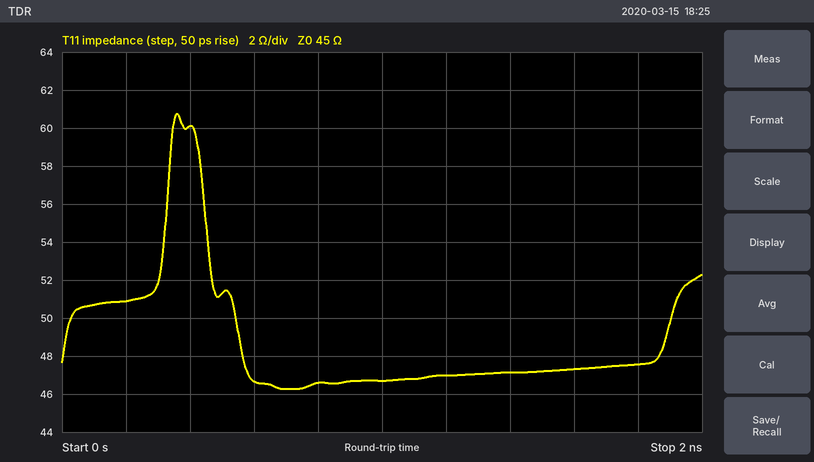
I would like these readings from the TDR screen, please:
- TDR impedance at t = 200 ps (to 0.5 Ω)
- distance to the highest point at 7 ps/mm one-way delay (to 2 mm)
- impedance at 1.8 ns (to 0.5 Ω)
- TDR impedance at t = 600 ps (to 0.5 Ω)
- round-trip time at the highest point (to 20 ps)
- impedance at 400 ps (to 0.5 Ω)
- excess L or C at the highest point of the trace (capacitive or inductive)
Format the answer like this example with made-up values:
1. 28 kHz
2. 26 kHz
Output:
1. 51.0 Ω
2. 26 mm
3. 47.5 Ω
4. 46.5 Ω
5. 360 ps
6. 60.0 Ω
7. inductive
